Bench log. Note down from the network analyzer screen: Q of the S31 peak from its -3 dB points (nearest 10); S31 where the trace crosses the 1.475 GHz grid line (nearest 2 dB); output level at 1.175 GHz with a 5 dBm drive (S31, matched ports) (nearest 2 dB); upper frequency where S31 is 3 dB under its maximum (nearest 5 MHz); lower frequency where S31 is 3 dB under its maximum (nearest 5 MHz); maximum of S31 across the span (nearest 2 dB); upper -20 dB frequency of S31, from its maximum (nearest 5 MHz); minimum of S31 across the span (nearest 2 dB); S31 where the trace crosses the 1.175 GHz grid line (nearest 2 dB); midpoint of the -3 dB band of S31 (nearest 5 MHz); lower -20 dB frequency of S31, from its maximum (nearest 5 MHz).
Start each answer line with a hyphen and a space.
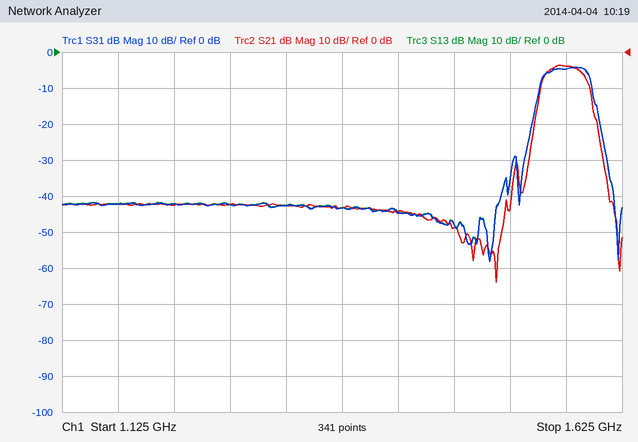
- 40
- -48 dB
- -38 dBm
- 1.595 GHz
- 1.555 GHz
- -4 dB
- 1.610 GHz
- -58 dB
- -42 dB
- 1.575 GHz
- 1.540 GHz
